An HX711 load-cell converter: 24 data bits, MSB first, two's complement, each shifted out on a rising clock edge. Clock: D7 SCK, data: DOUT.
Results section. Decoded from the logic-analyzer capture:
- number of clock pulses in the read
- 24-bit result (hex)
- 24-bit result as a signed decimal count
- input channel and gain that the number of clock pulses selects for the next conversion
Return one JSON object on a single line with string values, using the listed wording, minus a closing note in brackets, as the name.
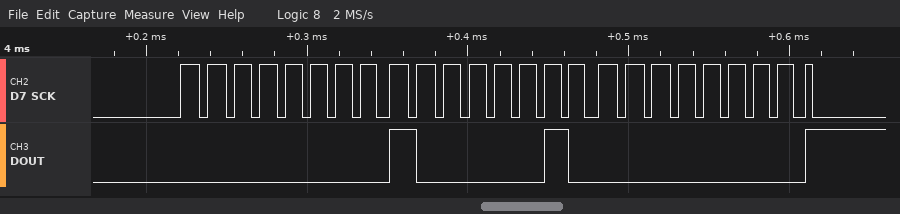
{"number of clock pulses in the read": "25", "24-bit result": "0x008200", "24-bit result as a signed decimal count": "33280", "input channel and gain that the number of clock pulses selects for the next conversion": "channel A, gain 128"}
